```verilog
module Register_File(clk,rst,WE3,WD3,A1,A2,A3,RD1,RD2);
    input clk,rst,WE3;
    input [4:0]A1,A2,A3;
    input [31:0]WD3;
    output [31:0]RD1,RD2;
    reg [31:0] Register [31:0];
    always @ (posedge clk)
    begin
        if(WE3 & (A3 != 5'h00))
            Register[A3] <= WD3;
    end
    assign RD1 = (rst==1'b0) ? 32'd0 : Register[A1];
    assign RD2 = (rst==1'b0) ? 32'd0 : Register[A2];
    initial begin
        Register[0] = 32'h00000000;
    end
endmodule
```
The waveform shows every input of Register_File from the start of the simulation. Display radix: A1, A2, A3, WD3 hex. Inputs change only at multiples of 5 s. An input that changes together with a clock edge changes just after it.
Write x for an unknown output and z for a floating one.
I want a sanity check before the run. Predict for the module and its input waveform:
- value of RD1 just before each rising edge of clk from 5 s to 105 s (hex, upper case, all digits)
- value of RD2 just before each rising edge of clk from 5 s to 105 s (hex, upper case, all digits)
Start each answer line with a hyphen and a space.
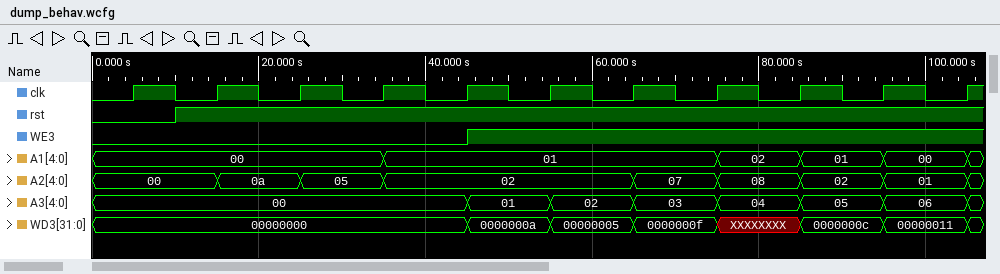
- 00000000, 00000000, 00000000, 00000000, x, x, 0000000A, 0000000A, 00000005, 0000000A, 00000000
- 00000000, 00000000, x, x, x, x, x, x, x, 00000005, 0000000A
